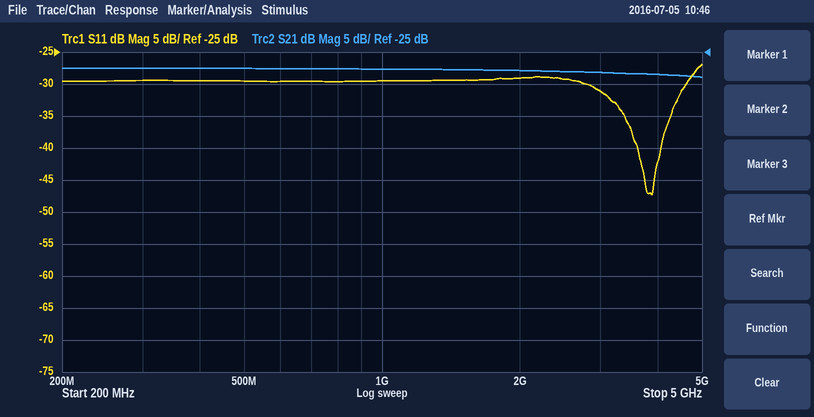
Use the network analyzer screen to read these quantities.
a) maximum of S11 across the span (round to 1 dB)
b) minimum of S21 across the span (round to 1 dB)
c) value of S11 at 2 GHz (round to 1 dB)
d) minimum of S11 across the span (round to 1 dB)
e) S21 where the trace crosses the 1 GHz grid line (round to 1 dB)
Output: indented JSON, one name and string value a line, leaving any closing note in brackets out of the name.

{
  "maximum of S11 across the span": "-27 dB",
  "minimum of S21 across the span": "-29 dB",
  "value of S11 at 2 GHz": "-29 dB",
  "minimum of S11 across the span": "-47 dB",
  "S21 where the trace crosses the 1 GHz grid line": "-28 dB"
}
